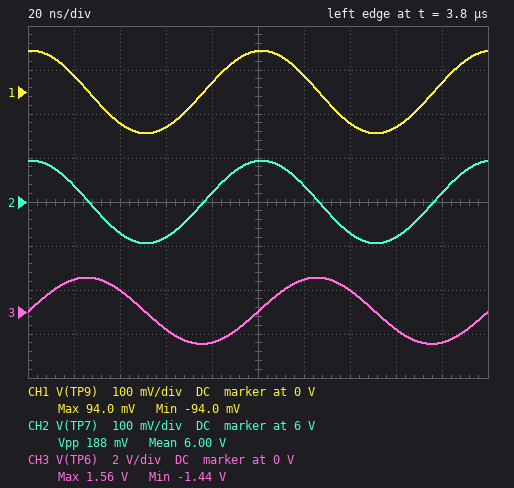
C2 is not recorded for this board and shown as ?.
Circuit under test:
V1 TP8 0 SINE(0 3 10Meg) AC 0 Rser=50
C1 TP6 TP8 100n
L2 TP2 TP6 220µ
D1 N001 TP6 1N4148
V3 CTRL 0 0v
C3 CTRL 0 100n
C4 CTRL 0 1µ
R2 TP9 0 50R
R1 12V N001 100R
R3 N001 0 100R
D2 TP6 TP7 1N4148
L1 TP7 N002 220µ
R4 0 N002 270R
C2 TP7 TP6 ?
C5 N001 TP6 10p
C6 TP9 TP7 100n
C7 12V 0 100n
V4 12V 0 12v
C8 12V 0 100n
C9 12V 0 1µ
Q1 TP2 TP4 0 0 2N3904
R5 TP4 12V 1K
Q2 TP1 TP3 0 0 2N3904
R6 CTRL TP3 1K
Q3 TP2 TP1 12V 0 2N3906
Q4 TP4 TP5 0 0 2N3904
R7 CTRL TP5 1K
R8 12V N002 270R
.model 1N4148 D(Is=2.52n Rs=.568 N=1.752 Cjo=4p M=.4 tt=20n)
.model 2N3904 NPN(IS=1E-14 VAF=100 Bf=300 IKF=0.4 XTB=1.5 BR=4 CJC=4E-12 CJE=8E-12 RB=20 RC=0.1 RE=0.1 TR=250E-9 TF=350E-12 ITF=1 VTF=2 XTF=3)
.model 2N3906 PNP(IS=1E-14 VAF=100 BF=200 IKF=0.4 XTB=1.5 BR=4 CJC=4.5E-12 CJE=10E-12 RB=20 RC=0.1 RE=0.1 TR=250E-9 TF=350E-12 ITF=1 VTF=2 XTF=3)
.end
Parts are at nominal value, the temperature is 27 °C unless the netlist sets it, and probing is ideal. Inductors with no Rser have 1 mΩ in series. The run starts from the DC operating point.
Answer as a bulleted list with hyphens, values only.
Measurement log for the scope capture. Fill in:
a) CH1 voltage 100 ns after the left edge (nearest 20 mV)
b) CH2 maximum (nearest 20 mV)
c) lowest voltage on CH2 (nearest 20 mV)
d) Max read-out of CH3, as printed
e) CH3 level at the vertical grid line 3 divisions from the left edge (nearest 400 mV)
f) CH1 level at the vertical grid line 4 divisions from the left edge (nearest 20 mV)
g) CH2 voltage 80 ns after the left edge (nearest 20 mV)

- 100 mV
- 6.10 V
- 5.90 V
- 1.56 V
- -800 mV
- 20 mV
- 6.02 V
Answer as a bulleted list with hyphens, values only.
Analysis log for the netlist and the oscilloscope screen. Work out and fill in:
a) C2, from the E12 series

- 18 pF
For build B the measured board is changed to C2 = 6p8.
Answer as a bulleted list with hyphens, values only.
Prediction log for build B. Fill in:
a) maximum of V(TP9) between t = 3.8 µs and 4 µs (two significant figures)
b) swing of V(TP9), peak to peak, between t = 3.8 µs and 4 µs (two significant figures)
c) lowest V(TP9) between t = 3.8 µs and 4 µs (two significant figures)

- 41 mV
- 82 mV
- -41 mV
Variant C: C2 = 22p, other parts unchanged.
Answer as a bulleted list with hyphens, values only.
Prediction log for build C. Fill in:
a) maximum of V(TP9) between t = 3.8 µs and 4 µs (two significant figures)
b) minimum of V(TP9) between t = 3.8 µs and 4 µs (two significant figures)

- 110 mV
- -110 mV
